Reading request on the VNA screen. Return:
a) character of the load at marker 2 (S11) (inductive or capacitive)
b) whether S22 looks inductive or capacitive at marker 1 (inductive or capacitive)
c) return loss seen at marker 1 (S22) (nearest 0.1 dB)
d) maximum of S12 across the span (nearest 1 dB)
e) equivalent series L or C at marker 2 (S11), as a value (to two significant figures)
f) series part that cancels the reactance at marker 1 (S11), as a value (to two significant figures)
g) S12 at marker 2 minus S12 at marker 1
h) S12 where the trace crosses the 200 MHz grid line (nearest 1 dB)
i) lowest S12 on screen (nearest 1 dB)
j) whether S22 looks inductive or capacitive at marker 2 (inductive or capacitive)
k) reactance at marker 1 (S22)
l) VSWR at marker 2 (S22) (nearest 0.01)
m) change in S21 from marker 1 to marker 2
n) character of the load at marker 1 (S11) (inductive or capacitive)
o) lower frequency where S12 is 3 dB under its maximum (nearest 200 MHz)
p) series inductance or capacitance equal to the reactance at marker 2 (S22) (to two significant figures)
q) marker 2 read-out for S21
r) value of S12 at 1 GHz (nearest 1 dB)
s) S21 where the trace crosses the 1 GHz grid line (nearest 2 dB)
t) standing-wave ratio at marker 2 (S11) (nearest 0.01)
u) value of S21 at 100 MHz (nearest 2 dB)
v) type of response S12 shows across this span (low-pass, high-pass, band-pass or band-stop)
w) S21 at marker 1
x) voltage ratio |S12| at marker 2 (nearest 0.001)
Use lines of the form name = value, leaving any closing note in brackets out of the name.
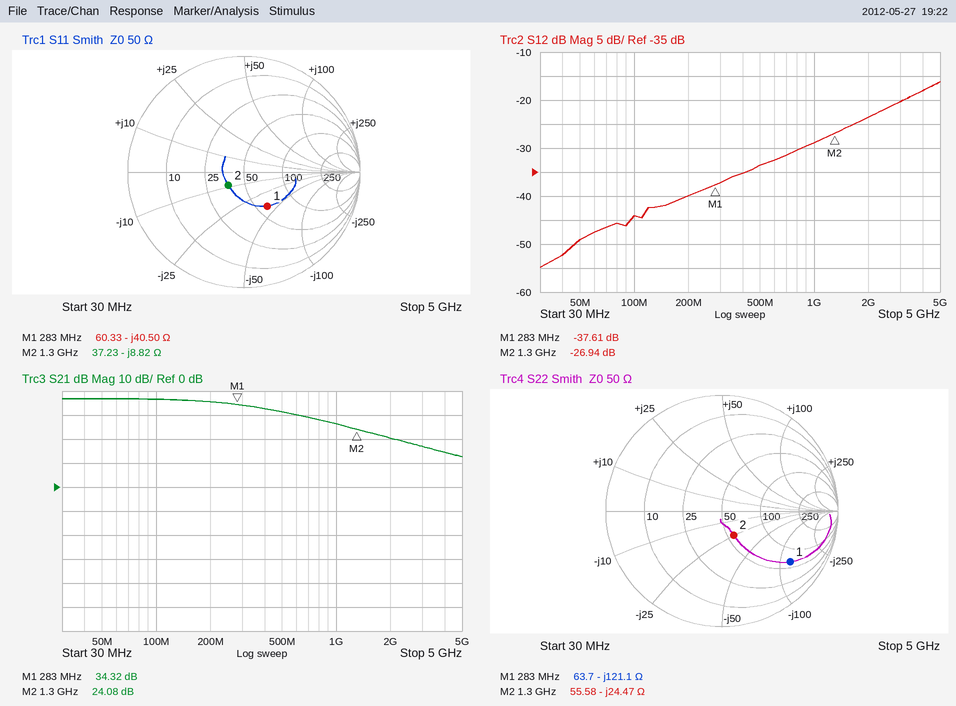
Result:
character of the load at marker 2 (S11) = capacitive
whether S22 looks inductive or capacitive at marker 1 = capacitive
return loss seen at marker 1 (S22) = 2.7 dB
maximum of S12 across the span = -16 dB
equivalent series L or C at marker 2 (S11), as a value = 14 pF
series part that cancels the reactance at marker 1 (S11), as a value = 23 nH
S12 at marker 2 minus S12 at marker 1 = 10.67 dB
S12 where the trace crosses the 200 MHz grid line = -40 dB
lowest S12 on screen = -55 dB
whether S22 looks inductive or capacitive at marker 2 = capacitive
reactance at marker 1 = -121.1 Ω
VSWR at marker 2 (S22) = 1.60
change in S21 from marker 1 to marker 2 = -10.24 dB
character of the load at marker 1 (S11) = capacitive
lower frequency where S12 is 3 dB under its maximum = 3.4 GHz
series inductance or capacitance equal to the reactance at marker 2 (S22) = 5.0 pF
marker 2 read-out for S21 = 24.08 dB
value of S12 at 1 GHz = -29 dB
S21 where the trace crosses the 1 GHz grid line = 26 dB
standing-wave ratio at marker 2 (S11) = 1.43
value of S21 at 100 MHz = 36 dB
type of response S12 shows across this span = high-pass
S21 at marker 1 = 34.32 dB
voltage ratio |S12| at marker 2 = 0.045
